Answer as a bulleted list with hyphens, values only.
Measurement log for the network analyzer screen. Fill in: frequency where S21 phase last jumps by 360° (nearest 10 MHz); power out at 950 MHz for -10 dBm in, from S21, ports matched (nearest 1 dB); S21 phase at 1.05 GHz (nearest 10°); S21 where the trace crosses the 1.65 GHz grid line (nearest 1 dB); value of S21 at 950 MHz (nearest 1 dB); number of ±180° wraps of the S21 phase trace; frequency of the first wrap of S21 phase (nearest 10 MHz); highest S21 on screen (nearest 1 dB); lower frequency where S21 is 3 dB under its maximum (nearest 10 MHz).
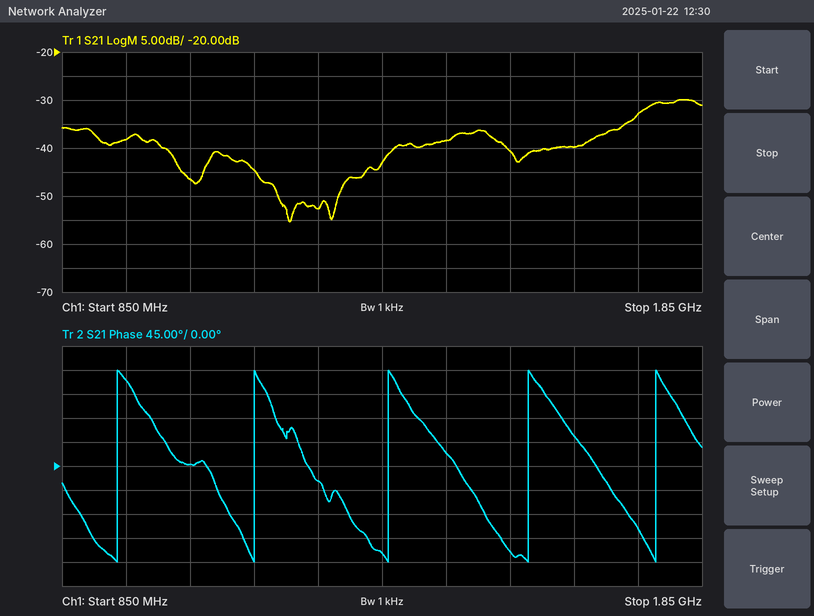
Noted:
- 1.78 GHz
- -48 dBm
- 0°
- -40 dB
- -38 dB
- 5
- 940 MHz
- -30 dB
- 1.75 GHz
